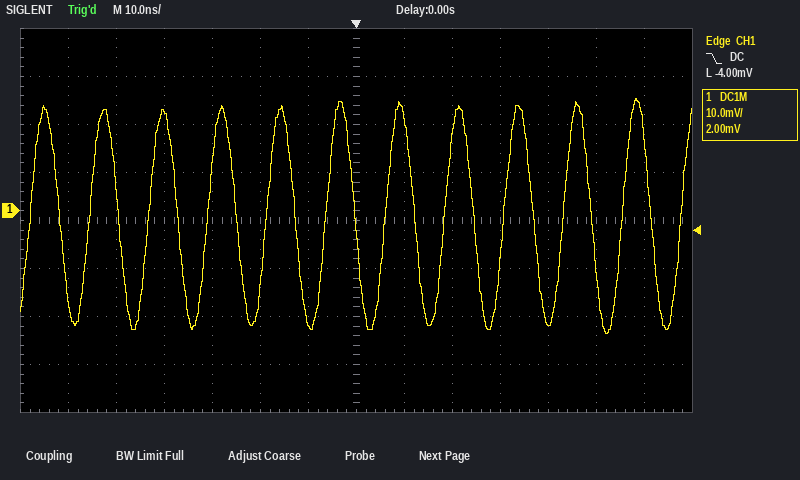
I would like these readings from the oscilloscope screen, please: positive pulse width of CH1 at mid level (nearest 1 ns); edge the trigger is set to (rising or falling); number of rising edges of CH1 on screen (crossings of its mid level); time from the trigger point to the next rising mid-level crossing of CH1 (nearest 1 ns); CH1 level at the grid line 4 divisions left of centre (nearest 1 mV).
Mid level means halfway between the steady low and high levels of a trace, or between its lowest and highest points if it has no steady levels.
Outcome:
6 ns
falling
12
6 ns
21 mV
